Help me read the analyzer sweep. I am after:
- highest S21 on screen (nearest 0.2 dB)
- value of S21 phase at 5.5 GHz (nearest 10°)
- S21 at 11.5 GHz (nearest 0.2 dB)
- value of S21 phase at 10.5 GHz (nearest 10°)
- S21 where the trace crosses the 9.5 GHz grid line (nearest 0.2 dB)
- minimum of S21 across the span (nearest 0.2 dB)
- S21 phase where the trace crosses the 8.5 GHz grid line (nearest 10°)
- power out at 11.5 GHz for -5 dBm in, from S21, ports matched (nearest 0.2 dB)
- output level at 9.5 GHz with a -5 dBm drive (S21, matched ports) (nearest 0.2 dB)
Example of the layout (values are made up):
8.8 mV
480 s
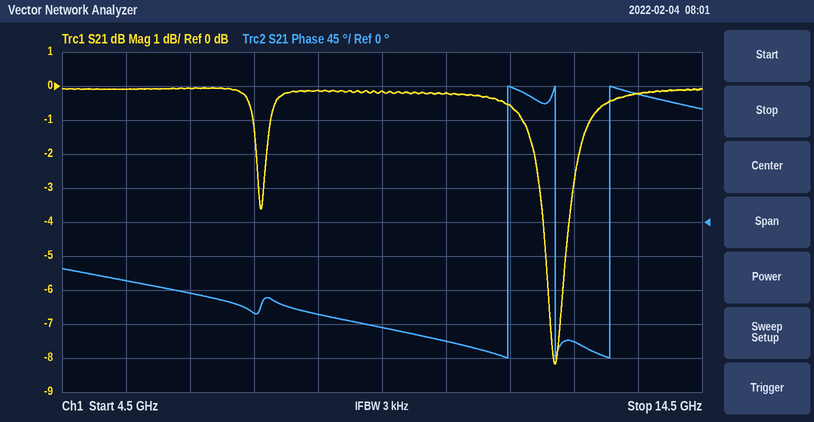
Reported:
0.0 dB
-80°
-0.6 dB
-160°
-0.2 dB
-8.2 dB
-120°
-5.6 dBm
-5.2 dBm
